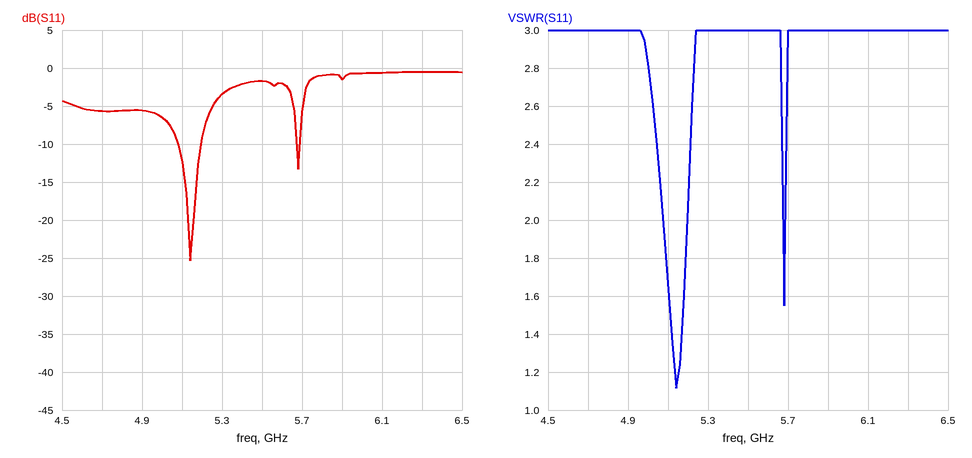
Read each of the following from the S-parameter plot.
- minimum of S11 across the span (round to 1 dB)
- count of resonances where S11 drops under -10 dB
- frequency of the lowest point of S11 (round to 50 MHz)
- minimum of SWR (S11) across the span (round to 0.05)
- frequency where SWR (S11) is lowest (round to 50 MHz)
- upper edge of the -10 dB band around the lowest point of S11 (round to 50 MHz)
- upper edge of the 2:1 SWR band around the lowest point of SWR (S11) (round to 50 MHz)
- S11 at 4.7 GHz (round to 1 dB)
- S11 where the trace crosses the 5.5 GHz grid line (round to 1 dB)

-25 dB
2
5.15 GHz
1.10
5.15 GHz
5.20 GHz
5.20 GHz
-6 dB
-2 dB
